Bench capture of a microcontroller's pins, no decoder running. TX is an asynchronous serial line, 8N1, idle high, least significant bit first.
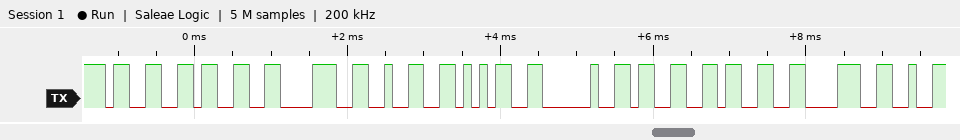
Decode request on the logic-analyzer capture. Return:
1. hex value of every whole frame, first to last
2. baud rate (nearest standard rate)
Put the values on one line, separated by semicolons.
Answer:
0x33 0x33 0x38 0x32 0x35 0x20 0x33 0x33 0x38; 9600 baud
